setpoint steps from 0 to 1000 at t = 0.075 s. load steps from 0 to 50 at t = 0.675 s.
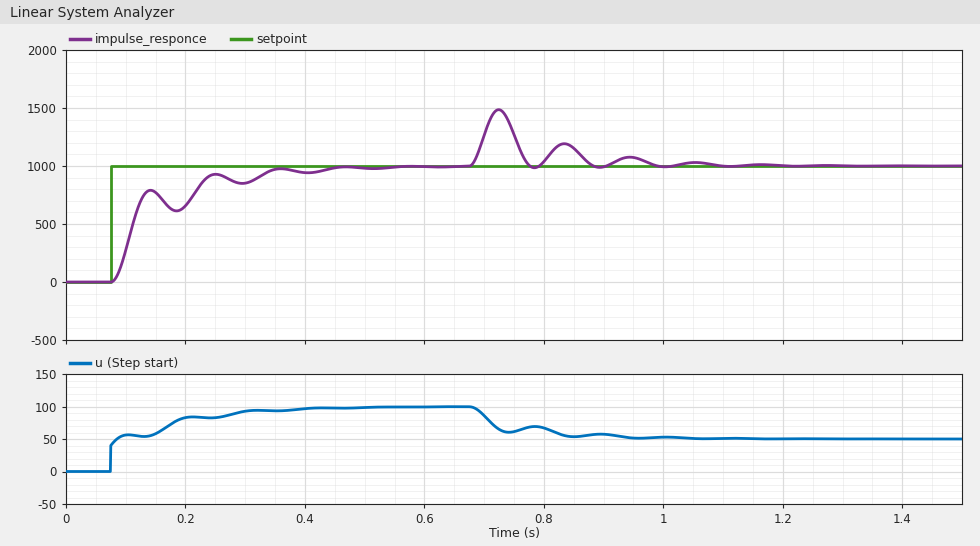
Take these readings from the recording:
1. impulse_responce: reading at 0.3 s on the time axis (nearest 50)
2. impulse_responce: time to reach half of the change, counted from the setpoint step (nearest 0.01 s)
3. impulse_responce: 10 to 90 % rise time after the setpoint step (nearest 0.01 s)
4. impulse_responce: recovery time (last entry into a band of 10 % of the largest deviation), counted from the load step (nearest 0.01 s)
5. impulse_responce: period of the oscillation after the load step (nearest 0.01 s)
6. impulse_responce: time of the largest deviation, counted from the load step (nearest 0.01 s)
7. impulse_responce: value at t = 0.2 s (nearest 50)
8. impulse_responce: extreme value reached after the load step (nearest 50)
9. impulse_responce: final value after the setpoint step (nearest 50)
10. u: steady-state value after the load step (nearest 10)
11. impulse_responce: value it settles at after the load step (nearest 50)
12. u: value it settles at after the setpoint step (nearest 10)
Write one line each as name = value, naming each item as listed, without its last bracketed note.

impulse_responce: reading at 0.3 s on the time axis = 850
impulse_responce: time to reach half of the change, counted from the setpoint step = 0.04 s
impulse_responce: 10 to 90 % rise time after the setpoint step = 0.15 s
impulse_responce: recovery time (last entry into a band of 10 % of the largest deviation), counted from the load step = 0.29 s
impulse_responce: period of the oscillation after the load step = 0.11 s
impulse_responce: time of the largest deviation, counted from the load step = 0.05 s
impulse_responce: value at t = 0.2 s = 650
impulse_responce: extreme value reached after the load step = 1500
impulse_responce: final value after the setpoint step = 1000
u: steady-state value after the load step = 50
impulse_responce: value it settles at after the load step = 1000
u: value it settles at after the setpoint step = 100
